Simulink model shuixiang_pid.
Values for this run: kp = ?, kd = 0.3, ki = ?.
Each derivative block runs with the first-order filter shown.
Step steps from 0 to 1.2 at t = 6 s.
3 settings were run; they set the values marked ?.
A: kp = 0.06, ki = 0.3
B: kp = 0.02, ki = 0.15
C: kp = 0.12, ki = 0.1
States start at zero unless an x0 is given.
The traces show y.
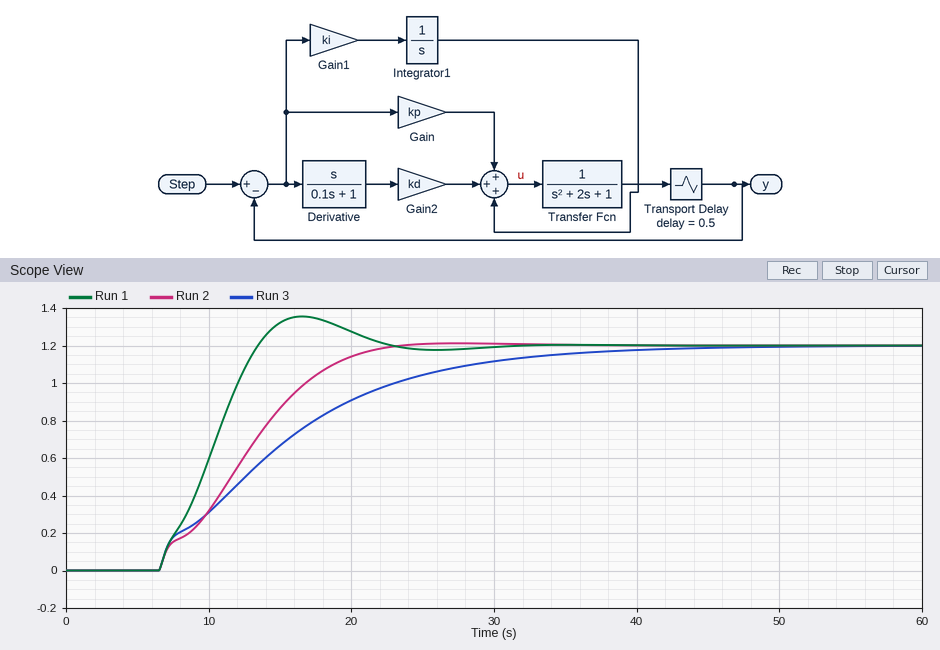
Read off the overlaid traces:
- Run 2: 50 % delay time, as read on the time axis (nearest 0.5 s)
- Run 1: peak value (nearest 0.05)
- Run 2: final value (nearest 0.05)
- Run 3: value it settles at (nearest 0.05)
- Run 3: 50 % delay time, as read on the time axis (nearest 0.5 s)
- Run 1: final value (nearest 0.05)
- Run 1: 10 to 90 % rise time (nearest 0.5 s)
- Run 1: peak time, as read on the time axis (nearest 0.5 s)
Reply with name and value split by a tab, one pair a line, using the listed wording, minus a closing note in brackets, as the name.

Run 2: 50 % delay time, as read on the time axis	12.5 s
Run 1: peak value	1.35
Run 2: final value	1.20
Run 3: value it settles at	1.20
Run 3: 50 % delay time, as read on the time axis	14.0 s
Run 1: final value	1.20
Run 1: 10 to 90 % rise time	5.5 s
Run 1: peak time, as read on the time axis	16.5 s
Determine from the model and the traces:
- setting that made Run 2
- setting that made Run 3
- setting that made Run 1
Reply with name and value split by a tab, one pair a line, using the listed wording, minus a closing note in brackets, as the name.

setting that made Run 2	B
setting that made Run 3	C
setting that made Run 1	A
